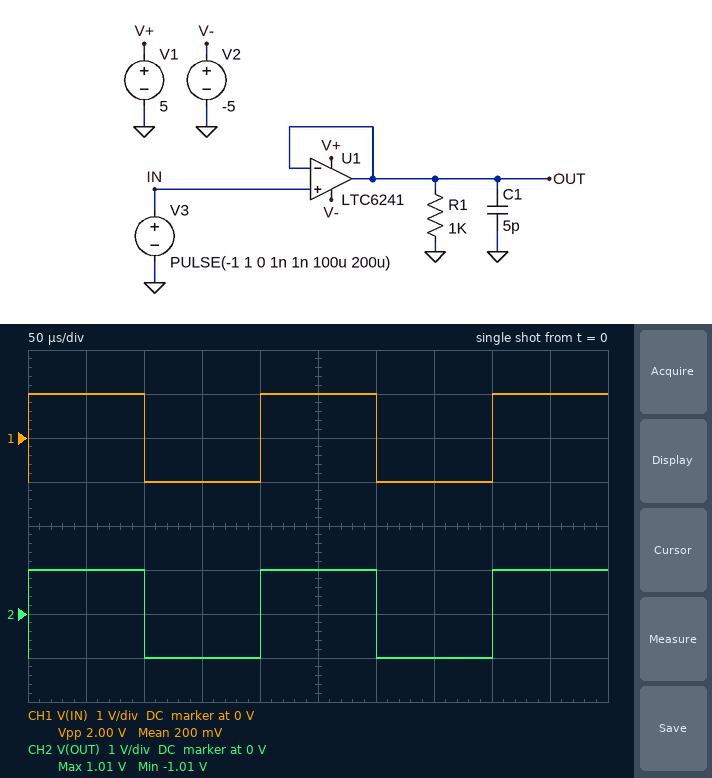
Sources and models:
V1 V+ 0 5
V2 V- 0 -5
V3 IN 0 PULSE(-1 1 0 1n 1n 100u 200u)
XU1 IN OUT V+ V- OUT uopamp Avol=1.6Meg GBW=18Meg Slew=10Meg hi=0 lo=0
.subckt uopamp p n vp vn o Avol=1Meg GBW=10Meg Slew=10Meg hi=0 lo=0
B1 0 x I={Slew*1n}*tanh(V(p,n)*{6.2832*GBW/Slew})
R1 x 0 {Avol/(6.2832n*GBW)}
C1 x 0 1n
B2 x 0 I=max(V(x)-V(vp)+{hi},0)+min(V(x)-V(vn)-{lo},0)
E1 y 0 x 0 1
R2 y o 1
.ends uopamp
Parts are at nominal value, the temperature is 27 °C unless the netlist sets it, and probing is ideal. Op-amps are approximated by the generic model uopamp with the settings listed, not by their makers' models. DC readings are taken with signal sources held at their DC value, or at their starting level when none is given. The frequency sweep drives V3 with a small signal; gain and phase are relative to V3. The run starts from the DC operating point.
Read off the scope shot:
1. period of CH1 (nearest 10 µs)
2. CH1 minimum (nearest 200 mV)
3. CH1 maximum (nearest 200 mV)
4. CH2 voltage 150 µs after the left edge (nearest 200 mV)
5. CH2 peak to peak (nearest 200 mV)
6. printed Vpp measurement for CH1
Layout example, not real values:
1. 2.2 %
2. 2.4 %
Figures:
1. 200 µs
2. -1.0 V
3. 1.0 V
4. -1.0 V
5. 2.0 V
6. 2.00 V
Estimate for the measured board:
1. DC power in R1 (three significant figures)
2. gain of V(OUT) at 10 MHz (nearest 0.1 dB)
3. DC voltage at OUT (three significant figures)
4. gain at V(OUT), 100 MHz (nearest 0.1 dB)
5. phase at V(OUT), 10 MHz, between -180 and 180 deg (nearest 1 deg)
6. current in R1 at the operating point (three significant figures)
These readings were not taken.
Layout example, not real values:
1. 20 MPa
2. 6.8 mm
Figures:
1. 1.00 mW
2. -1.2 dB
3. -1.00 V
4. -15.0 dB
5. -29 deg
6. 1.00 mA
